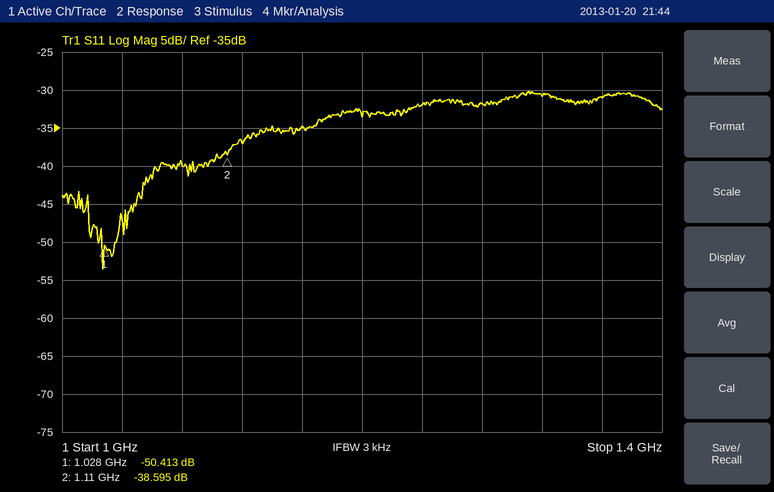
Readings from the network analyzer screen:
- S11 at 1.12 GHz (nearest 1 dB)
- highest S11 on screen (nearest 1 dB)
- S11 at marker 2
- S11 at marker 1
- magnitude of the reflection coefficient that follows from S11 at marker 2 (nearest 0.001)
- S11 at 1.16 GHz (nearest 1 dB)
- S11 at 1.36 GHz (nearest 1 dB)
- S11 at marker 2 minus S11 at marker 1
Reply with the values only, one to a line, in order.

-37 dB
-30 dB
-38.595 dB
-50.413 dB
0.012
-35 dB
-31 dB
11.818 dB
